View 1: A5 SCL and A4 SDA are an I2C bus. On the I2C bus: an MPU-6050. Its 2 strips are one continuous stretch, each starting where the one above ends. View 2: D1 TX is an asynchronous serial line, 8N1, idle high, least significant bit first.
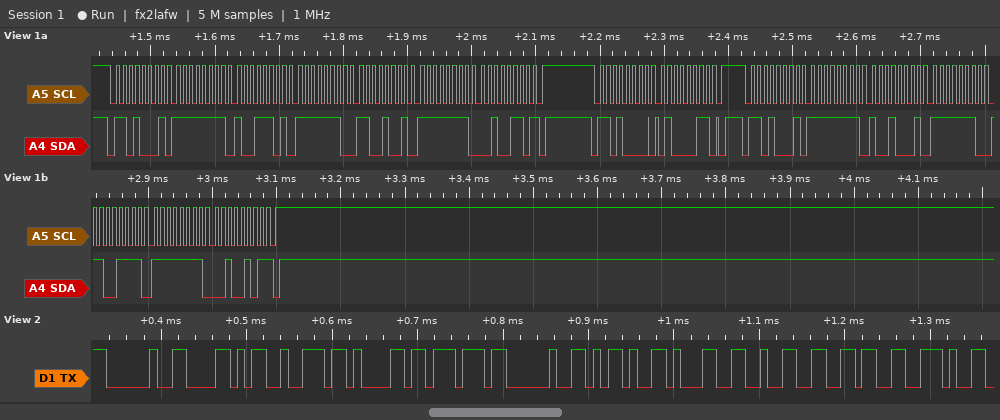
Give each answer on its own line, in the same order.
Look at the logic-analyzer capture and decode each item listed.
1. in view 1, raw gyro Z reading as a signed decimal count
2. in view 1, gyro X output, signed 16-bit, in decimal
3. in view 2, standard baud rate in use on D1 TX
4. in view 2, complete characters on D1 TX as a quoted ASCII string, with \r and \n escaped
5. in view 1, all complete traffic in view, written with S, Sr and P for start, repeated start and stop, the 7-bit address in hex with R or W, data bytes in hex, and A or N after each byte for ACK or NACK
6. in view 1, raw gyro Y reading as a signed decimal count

-219
-111
115200 baud
" Xraw -126."
S 68R A FF A 9D A FE A C9 A FF A 26 N P S 68W A 43 A P S 68R A FF A 91 A FE A CF A FF A 25 N P
-305
